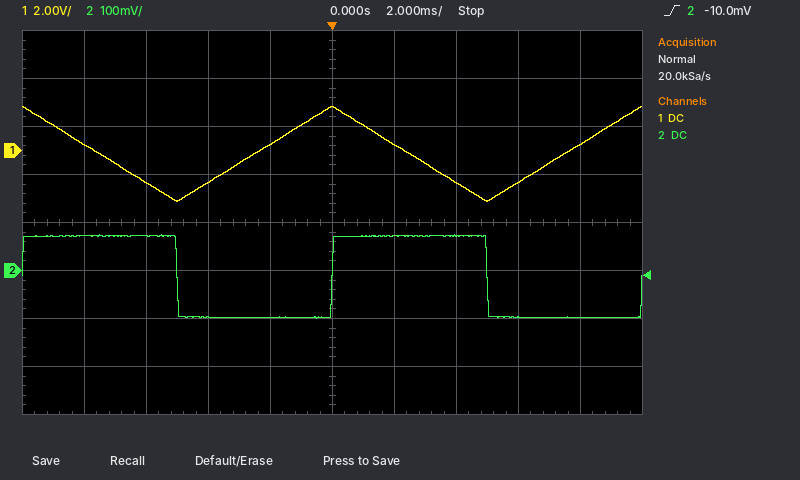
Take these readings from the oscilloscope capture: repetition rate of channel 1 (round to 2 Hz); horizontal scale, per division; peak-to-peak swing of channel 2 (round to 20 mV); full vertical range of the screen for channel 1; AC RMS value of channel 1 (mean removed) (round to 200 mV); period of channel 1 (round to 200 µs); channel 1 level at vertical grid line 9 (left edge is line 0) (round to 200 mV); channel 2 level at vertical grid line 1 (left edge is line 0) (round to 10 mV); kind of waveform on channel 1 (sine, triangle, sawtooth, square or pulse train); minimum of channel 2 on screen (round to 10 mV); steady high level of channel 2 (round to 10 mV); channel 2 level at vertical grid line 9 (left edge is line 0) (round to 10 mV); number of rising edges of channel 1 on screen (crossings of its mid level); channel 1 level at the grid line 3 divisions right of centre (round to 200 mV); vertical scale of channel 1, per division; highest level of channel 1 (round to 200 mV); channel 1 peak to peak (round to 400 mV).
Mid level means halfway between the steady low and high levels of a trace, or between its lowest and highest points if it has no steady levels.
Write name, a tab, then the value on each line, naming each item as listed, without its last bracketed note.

repetition rate of channel 1	100 Hz
horizontal scale, per division	2 ms
peak-to-peak swing of channel 2	180 mV
full vertical range of the screen for channel 1	16 V
AC RMS value of channel 1 (mean removed)	1.2 V
period of channel 1	10.0 ms
channel 1 level at vertical grid line 9 (left edge is line 0)	200 mV
channel 2 level at vertical grid line 1 (left edge is line 0)	70 mV
kind of waveform on channel 1	triangle
minimum of channel 2 on screen	-100 mV
steady high level of channel 2	70 mV
channel 2 level at vertical grid line 9 (left edge is line 0)	-100 mV
number of rising edges of channel 1 on screen	2
channel 1 level at the grid line 3 divisions right of centre	-1.4 V
vertical scale of channel 1, per division	2 V
highest level of channel 1	1.8 V
channel 1 peak to peak	4.0 V
